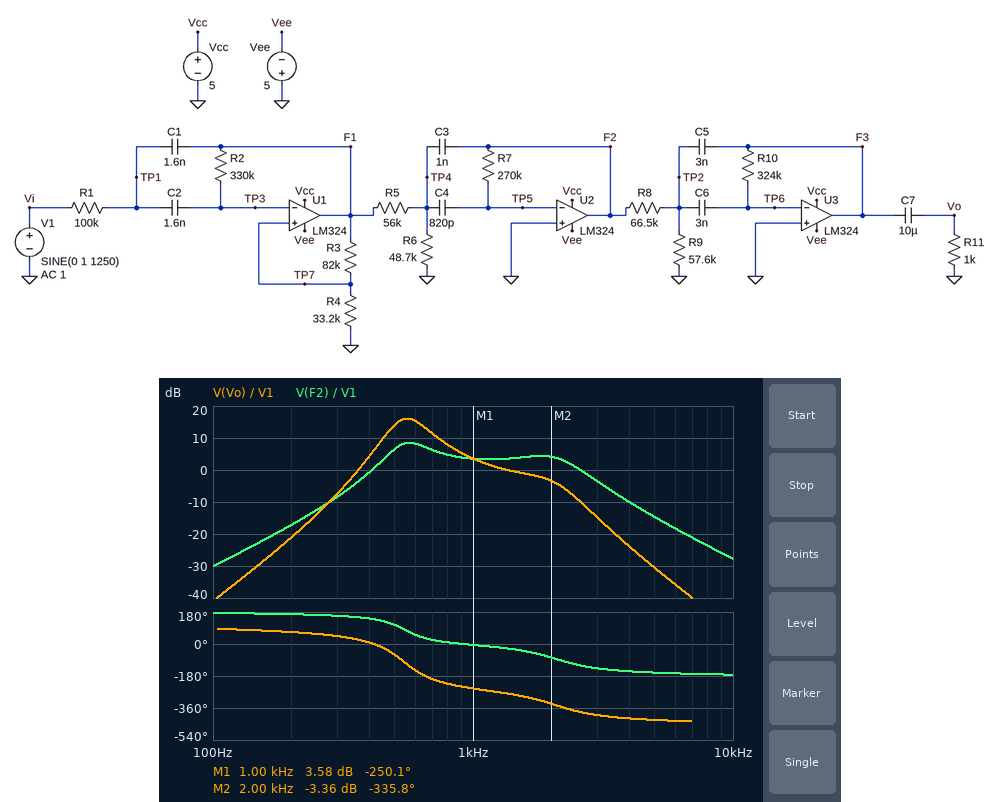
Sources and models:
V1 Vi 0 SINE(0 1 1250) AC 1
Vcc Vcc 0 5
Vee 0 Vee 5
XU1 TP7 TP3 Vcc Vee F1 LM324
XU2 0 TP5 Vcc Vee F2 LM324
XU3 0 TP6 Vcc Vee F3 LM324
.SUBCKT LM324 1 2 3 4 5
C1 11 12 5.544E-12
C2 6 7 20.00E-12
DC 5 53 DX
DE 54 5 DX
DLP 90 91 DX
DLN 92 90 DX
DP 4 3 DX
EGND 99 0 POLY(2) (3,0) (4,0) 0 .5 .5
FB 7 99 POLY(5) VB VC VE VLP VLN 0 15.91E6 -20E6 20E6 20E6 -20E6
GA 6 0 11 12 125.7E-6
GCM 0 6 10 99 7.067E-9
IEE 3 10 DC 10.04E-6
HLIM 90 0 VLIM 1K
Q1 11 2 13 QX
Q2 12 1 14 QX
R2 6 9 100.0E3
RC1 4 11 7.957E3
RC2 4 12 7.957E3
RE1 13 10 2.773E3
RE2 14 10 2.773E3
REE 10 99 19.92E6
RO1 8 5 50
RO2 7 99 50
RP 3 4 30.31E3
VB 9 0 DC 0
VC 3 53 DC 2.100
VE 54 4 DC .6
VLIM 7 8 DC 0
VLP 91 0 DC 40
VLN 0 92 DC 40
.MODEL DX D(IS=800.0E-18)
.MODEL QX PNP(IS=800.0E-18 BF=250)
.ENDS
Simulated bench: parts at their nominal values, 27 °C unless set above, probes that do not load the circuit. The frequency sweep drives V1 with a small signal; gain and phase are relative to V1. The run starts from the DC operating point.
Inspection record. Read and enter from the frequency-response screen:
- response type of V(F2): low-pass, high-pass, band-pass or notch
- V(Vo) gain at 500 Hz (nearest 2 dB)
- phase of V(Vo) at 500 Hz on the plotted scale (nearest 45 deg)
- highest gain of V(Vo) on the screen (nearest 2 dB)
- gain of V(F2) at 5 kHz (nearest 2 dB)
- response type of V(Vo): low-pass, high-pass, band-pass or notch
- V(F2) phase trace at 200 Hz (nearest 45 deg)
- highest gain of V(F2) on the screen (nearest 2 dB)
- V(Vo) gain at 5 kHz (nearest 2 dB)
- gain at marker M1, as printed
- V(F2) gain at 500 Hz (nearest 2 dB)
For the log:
band-pass
14 dB
-45 deg
16 dB
-14 dB
band-pass
180 deg
8 dB
-30 dB
3.58 dB
6 dB
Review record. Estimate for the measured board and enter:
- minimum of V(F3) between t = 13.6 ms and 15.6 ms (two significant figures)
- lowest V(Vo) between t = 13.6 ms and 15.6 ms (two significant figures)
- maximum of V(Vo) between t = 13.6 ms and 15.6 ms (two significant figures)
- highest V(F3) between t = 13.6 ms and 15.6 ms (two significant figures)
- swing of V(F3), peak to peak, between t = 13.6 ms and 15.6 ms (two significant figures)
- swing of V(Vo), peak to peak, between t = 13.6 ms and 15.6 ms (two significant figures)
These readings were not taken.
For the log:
-1.1 V
-1.1 V
1.1 V
1.1 V
2.2 V
2.2 V
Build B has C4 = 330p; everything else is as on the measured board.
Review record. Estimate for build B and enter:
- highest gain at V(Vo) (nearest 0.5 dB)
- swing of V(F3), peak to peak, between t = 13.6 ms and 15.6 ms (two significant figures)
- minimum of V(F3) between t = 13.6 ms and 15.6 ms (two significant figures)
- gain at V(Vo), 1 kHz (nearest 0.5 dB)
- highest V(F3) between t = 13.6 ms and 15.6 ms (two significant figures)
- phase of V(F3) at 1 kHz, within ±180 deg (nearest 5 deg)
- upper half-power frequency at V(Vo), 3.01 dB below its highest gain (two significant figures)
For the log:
8.0 dB
730 mV
-370 mV
-5.5 dB
360 mV
115 deg
650 Hz
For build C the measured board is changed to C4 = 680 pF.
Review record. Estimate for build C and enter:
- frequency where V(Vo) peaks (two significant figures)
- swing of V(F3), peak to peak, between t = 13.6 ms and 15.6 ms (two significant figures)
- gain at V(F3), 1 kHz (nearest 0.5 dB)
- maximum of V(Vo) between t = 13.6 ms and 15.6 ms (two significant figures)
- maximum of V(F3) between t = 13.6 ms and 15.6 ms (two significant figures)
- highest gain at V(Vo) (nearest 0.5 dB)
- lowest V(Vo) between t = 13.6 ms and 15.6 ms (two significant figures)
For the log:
560 Hz
1.7 V
1.5 dB
860 mV
850 mV
14.5 dB
-860 mV
